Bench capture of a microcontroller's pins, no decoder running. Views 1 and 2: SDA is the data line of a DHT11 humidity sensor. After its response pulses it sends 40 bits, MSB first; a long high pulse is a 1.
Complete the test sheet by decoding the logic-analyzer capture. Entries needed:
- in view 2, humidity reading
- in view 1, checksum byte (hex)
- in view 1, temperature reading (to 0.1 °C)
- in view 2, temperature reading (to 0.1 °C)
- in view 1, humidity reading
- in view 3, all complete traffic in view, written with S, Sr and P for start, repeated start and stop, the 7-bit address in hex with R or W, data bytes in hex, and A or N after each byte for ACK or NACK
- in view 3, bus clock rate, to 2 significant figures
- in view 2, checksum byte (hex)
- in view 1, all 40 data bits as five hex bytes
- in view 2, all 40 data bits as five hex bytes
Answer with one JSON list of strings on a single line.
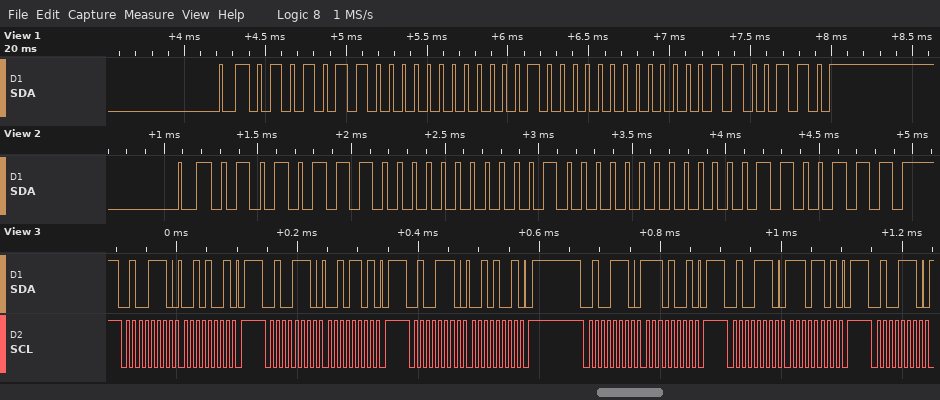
["87 %", "0x66", "16.0 °C", "16.0 °C", "86 %", "S 27W A 29 A P S 27W A 2D A P S 27W A 29 A P S 27W A E9 A P S 27W A ED A P S 27W A", "100 kHz", "0x67", "56 00 10 00 66", "57 00 10 00 67"]
